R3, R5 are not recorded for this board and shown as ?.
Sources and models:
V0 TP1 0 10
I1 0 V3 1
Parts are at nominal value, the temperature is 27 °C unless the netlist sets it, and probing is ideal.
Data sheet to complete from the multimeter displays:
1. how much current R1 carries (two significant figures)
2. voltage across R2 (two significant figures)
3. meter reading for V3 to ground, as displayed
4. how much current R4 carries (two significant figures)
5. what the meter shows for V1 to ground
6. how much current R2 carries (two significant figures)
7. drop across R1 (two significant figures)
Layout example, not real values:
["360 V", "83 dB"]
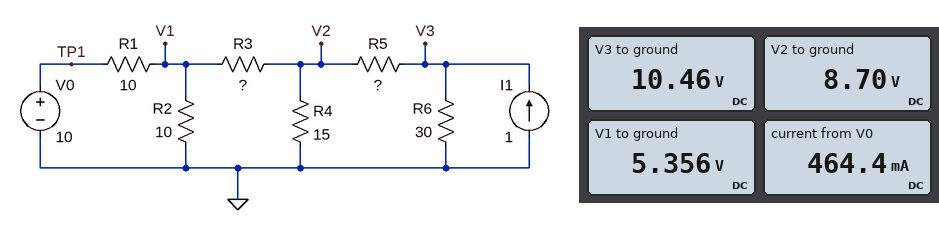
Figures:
["460 mA", "5.4 V", "10.46 V", "580 mA", "5.356 V", "540 mA", "4.6 V"]
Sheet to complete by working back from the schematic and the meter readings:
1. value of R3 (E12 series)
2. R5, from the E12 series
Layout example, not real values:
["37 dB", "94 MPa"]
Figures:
["47 Ω", "2.7 Ω"]
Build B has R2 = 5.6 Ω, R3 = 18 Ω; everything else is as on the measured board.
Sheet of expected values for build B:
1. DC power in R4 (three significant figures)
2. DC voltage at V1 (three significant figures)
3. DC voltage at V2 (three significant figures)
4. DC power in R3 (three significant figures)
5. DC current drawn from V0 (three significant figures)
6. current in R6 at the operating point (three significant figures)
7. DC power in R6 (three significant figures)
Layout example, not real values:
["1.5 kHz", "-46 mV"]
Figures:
["3.80 W", "4.25 V", "7.55 V", "605 mW", "575 mA", "313 mA", "2.95 W"]
